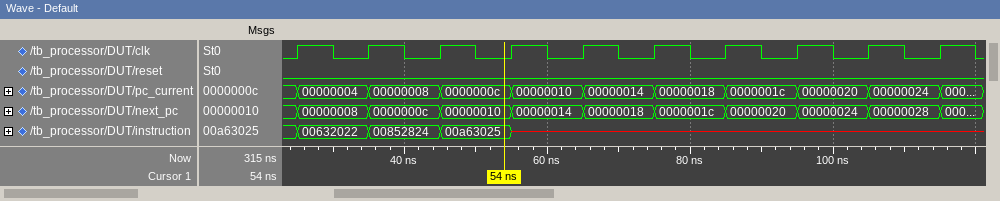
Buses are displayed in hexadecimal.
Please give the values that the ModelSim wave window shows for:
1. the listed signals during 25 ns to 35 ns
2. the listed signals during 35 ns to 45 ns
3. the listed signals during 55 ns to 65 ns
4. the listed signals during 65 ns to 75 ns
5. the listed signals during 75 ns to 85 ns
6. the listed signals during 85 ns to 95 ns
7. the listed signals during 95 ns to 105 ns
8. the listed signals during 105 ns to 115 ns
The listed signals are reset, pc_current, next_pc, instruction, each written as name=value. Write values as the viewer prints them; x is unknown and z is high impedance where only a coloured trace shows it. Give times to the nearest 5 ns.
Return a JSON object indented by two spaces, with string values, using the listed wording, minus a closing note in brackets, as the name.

{
  "the listed signals during 25 ns to 35 ns": "reset=0, pc_current=00000004, next_pc=00000008, instruction=00632022",
  "the listed signals during 35 ns to 45 ns": "reset=0, pc_current=00000008, next_pc=0000000c, instruction=00852824",
  "the listed signals during 55 ns to 65 ns": "reset=0, pc_current=00000010, next_pc=00000014, instruction=x",
  "the listed signals during 65 ns to 75 ns": "reset=0, pc_current=00000014, next_pc=00000018, instruction=x",
  "the listed signals during 75 ns to 85 ns": "reset=0, pc_current=00000018, next_pc=0000001c, instruction=x",
  "the listed signals during 85 ns to 95 ns": "reset=0, pc_current=0000001c, next_pc=00000020, instruction=x",
  "the listed signals during 95 ns to 105 ns": "reset=0, pc_current=00000020, next_pc=00000024, instruction=x",
  "the listed signals during 105 ns to 115 ns": "reset=0, pc_current=00000024, next_pc=00000028, instruction=x"
}
